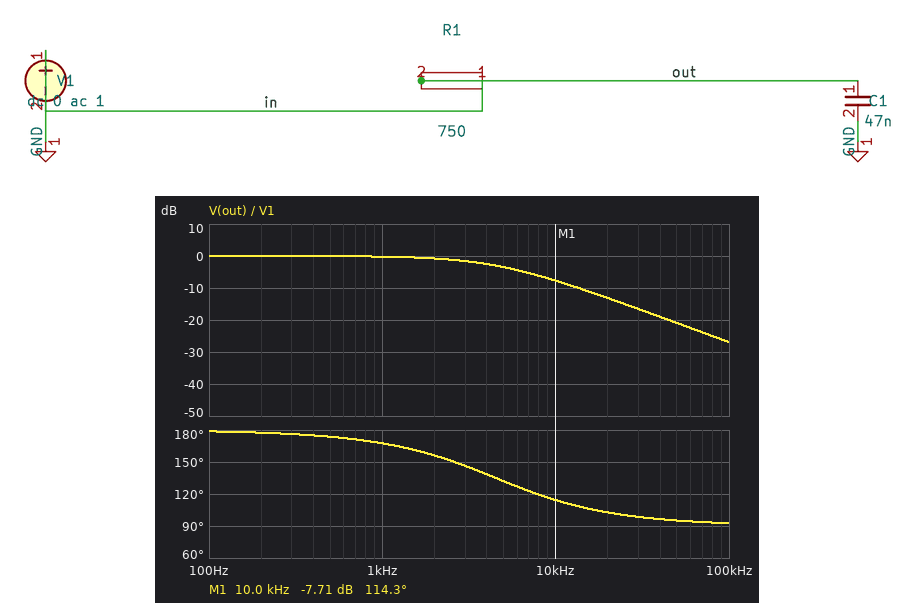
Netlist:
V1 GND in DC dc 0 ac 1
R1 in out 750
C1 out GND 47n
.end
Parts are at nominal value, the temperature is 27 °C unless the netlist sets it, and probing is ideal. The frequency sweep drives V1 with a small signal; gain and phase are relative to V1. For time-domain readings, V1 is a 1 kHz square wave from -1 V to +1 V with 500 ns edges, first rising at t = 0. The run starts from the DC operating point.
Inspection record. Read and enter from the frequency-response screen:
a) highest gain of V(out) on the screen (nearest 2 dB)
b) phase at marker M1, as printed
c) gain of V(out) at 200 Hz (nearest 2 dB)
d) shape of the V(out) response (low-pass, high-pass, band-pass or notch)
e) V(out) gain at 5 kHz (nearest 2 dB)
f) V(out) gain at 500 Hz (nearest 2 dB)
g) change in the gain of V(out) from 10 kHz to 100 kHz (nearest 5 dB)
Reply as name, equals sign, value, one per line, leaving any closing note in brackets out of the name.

highest gain of V(out) on the screen = 0 dB
phase at marker M1, as printed = 114.3 deg
gain of V(out) at 200 Hz = 0 dB
shape of the V(out) response = low-pass
V(out) gain at 5 kHz = -4 dB
V(out) gain at 500 Hz = 0 dB
change in the gain of V(out) from 10 kHz to 100 kHz = -20 dB
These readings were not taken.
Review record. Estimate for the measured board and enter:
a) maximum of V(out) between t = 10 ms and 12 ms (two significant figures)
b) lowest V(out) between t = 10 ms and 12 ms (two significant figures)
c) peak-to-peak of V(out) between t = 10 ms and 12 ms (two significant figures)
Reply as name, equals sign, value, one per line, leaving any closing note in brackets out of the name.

maximum of V(out) between t = 10 ms and 12 ms = 1.0 V
lowest V(out) between t = 10 ms and 12 ms = -1.0 V
peak-to-peak of V(out) between t = 10 ms and 12 ms = 2.0 V
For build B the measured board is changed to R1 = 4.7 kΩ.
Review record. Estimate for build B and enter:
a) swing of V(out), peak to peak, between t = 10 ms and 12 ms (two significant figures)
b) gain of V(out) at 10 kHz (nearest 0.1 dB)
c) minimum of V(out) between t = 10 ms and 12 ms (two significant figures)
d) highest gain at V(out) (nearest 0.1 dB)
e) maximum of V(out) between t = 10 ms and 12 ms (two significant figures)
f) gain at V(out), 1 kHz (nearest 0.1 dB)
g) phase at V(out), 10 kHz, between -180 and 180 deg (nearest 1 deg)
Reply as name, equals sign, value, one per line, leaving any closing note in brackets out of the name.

swing of V(out), peak to peak, between t = 10 ms and 12 ms = 1.6 V
gain of V(out) at 10 kHz = -22.9 dB
minimum of V(out) between t = 10 ms and 12 ms = -810 mV
highest gain at V(out) = 0 dB
maximum of V(out) between t = 10 ms and 12 ms = 810 mV
gain at V(out), 1 kHz = -4.7 dB
phase at V(out), 10 kHz, between -180 and 180 deg = 94 deg
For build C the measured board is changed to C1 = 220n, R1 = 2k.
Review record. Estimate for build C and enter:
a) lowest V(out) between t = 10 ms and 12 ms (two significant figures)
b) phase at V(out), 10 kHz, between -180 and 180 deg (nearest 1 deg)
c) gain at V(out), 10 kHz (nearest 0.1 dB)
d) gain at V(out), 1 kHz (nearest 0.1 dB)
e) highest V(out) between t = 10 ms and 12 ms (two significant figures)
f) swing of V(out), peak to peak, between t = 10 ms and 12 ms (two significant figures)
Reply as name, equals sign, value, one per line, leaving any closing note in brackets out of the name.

lowest V(out) between t = 10 ms and 12 ms = -510 mV
phase at V(out), 10 kHz, between -180 and 180 deg = 92 deg
gain at V(out), 10 kHz = -28.8 dB
gain at V(out), 1 kHz = -9.4 dB
highest V(out) between t = 10 ms and 12 ms = 510 mV
swing of V(out), peak to peak, between t = 10 ms and 12 ms = 1.0 V
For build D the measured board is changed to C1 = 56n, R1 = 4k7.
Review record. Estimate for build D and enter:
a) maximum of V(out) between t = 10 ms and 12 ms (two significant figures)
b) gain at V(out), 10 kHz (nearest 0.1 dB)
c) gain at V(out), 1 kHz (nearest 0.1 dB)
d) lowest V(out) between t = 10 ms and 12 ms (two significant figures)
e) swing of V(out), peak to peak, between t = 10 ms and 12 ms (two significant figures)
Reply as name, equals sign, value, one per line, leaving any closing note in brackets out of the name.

maximum of V(out) between t = 10 ms and 12 ms = 740 mV
gain at V(out), 10 kHz = -24.4 dB
gain at V(out), 1 kHz = -5.7 dB
lowest V(out) between t = 10 ms and 12 ms = -740 mV
swing of V(out), peak to peak, between t = 10 ms and 12 ms = 1.5 V
